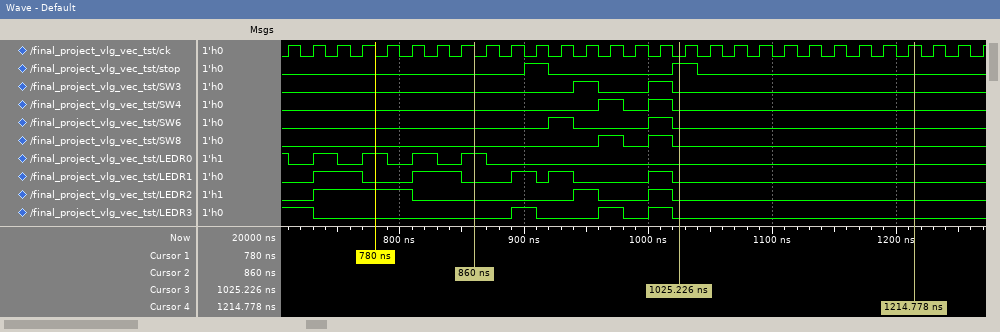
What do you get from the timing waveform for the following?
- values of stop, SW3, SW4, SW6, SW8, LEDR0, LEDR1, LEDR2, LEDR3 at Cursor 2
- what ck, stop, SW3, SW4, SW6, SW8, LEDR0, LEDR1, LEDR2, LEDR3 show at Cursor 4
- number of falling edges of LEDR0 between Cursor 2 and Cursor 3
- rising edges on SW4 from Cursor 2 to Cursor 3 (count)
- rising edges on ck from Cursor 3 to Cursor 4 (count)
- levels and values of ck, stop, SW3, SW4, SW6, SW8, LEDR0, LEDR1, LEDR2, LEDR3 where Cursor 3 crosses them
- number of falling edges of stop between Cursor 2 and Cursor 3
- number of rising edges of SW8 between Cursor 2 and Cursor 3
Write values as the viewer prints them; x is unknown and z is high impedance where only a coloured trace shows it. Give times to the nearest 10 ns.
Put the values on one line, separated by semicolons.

stop=0, SW3=0, SW4=0, SW6=0, SW8=0, LEDR0=1, LEDR1=0, LEDR2=0, LEDR3=0; ck=1, stop=0, SW3=0, SW4=0, SW6=0, SW8=0, LEDR0=0, LEDR1=0, LEDR2=0, LEDR3=0; 1; 2; 10; ck=0, stop=1, SW3=0, SW4=0, SW6=0, SW8=0, LEDR0=0, LEDR1=0, LEDR2=0, LEDR3=0; 1; 2
